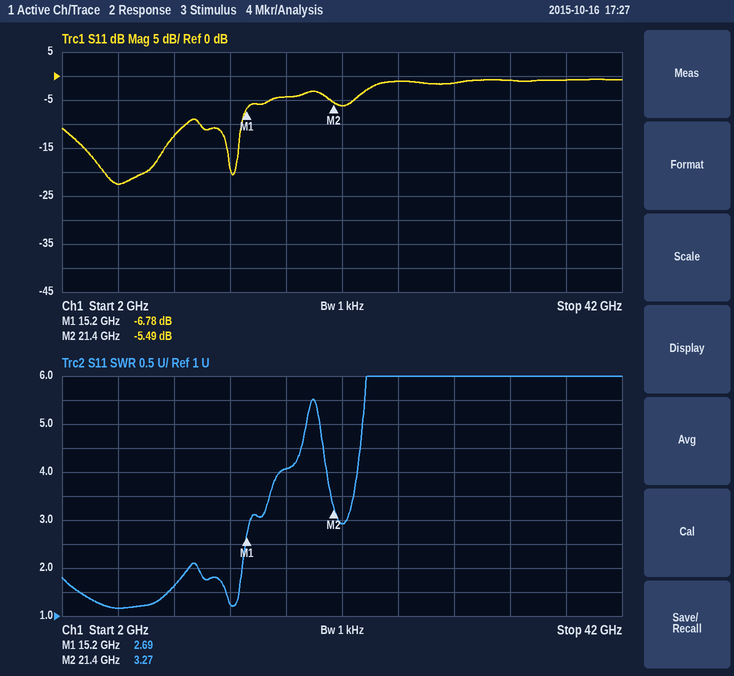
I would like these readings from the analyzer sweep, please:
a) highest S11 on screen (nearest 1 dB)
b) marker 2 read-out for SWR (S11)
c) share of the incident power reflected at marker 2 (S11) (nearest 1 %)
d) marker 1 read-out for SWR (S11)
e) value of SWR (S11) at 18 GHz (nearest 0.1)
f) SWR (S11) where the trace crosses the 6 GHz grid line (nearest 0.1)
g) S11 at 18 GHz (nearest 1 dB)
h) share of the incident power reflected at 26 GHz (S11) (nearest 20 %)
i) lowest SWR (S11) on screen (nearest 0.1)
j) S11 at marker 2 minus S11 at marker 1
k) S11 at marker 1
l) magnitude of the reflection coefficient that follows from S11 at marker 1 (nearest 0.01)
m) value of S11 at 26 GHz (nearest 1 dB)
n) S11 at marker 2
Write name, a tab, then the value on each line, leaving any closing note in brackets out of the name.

highest S11 on screen	-1 dB
marker 2 read-out for SWR	3.27
share of the incident power reflected at marker 2 (S11)	28 %
marker 1 read-out for SWR	2.69
value of SWR (S11) at 18 GHz	4.1
SWR (S11) where the trace crosses the 6 GHz grid line	1.2
S11 at 18 GHz	-4 dB
share of the incident power reflected at 26 GHz (S11)	80 %
lowest SWR (S11) on screen	1.2
S11 at marker 2 minus S11 at marker 1	1.29 dB
S11 at marker 1	-6.78 dB
magnitude of the reflection coefficient that follows from S11 at marker 1	0.46
value of S11 at 26 GHz	-1 dB
S11 at marker 2	-5.49 dB
